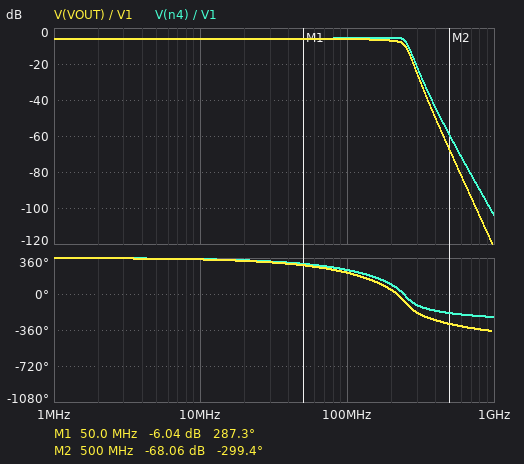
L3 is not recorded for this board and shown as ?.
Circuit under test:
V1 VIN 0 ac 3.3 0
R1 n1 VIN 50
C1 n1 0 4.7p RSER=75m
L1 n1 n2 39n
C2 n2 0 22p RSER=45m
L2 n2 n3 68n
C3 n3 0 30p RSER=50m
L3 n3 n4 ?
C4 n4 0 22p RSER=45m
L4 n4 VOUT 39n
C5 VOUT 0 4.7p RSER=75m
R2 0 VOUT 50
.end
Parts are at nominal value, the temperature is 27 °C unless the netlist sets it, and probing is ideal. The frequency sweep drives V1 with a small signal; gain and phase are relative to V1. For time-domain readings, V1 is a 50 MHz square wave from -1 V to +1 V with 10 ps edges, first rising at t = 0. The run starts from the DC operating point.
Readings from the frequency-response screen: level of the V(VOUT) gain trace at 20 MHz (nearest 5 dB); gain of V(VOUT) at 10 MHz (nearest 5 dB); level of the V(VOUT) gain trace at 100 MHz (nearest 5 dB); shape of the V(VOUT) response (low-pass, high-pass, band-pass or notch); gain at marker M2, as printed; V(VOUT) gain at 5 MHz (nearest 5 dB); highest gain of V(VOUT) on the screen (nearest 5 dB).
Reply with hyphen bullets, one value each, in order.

- -5 dB
- -5 dB
- -5 dB
- low-pass
- -68.06 dB
- -5 dB
- -5 dB
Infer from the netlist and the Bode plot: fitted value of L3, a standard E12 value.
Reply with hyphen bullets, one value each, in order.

- 47 nH
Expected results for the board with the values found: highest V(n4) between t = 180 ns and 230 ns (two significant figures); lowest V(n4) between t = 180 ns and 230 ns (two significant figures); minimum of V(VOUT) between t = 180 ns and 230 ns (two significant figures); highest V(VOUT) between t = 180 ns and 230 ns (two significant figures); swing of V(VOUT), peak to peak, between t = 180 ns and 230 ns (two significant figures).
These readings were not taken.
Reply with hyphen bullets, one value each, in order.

- 720 mV
- -720 mV
- -670 mV
- 670 mV
- 1.3 V
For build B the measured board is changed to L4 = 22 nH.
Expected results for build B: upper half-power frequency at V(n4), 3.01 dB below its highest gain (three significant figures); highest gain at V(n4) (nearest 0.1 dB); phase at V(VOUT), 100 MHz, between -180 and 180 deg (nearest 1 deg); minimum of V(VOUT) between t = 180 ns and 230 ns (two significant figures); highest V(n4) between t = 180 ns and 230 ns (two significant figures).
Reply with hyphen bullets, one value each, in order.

- 235 MHz
- -6.0 dB
- -141 deg
- -650 mV
- 650 mV
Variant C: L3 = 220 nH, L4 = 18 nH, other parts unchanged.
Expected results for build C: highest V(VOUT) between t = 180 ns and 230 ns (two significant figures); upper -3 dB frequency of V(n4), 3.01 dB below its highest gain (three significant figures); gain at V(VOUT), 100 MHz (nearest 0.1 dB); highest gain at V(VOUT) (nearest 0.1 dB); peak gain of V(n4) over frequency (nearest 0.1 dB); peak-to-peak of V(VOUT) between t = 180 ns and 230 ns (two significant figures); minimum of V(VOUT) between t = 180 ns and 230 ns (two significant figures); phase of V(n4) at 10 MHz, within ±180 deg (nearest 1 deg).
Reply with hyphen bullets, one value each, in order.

- 510 mV
- 91.0 MHz
- -9.7 dB
- -6.0 dB
- -6.0 dB
- 1.0 V
- -510 mV
- -19 deg
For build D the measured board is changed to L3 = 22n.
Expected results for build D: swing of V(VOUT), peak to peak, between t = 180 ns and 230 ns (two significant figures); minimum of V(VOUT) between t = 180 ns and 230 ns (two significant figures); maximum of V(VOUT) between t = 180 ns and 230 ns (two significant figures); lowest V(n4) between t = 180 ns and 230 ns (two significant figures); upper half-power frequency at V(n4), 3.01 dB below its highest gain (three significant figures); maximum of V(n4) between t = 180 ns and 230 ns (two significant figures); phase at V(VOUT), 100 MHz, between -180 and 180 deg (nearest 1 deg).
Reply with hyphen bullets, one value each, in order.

- 1.1 V
- -570 mV
- 570 mV
- -610 mV
- 212 MHz
- 610 mV
- -139 deg
